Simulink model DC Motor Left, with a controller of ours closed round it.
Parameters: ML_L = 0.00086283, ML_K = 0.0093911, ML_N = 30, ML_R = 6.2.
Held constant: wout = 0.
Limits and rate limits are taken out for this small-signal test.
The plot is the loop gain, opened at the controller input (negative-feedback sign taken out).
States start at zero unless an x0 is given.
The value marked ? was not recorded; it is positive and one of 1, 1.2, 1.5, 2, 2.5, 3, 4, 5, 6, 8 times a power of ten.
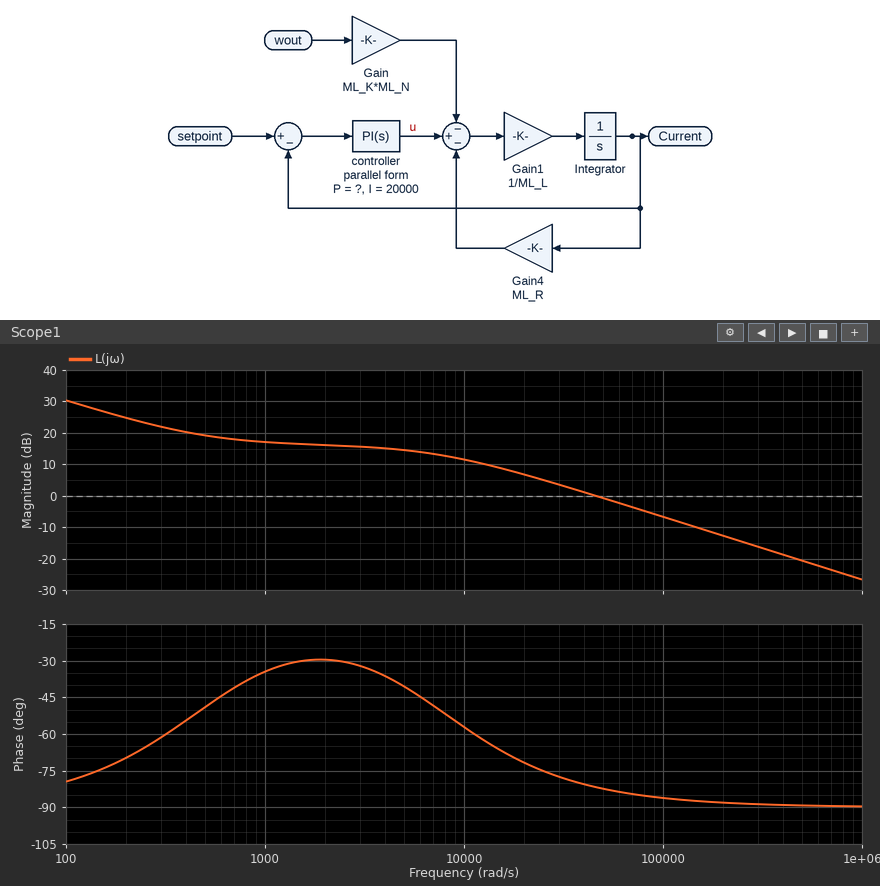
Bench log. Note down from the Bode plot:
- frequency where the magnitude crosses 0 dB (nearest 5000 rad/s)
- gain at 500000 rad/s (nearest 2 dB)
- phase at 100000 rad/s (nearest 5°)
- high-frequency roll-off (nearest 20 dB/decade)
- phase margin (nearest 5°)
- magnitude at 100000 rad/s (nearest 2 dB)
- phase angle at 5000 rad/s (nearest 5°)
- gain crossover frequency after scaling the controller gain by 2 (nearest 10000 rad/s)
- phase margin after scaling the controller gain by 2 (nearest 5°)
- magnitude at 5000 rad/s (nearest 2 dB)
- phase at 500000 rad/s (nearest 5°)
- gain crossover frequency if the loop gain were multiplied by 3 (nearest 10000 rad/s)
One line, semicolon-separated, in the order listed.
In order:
45000 rad/s; -20 dB; -85°; -20 dB/decade; 100°; -6 dB; -40°; 90000 rad/s; 95°; 14 dB; -90°; 140000 rad/s
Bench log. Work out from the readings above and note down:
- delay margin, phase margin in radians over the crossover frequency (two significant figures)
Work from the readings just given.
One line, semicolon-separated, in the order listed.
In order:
0.000039 s
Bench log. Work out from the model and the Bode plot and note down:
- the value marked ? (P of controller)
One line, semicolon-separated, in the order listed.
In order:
40
